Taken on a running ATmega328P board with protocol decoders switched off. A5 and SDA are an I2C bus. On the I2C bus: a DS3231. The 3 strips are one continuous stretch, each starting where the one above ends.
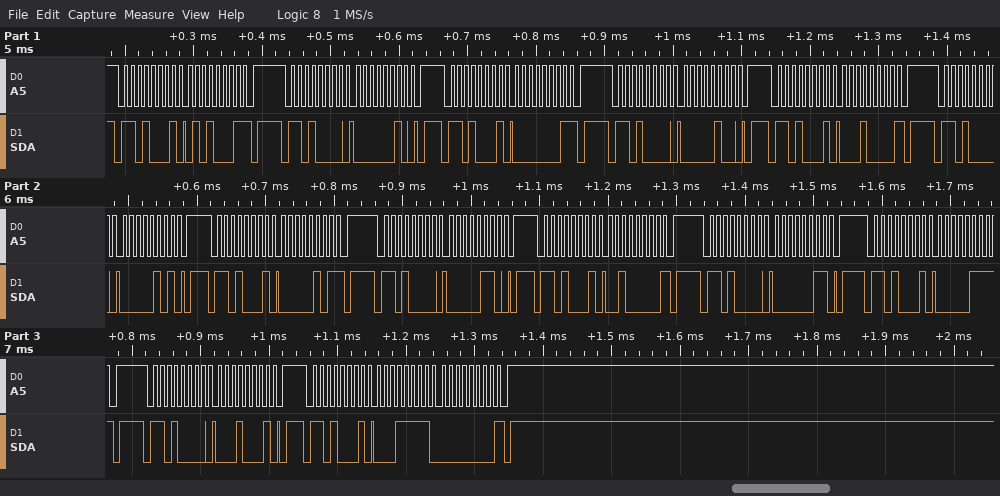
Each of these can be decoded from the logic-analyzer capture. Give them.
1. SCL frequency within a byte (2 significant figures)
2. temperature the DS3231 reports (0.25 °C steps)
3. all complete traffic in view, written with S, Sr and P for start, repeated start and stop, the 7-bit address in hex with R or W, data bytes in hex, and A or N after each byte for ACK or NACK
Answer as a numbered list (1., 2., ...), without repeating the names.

1. 100 kHz
2. 31.00 °C
3. S 68R A 51 N P S 68W A 02 A P S 68R A 01 N P S 68W A 04 A P S 68R A 10 N P S 68W A 05 A P S 68R A 05 N P S 68W A 06 A P S 68R A 20 N P S 68W A 03 A P S 68R A 07 N P S 68W A 11 A P S 68R A 1F A 00 N P
